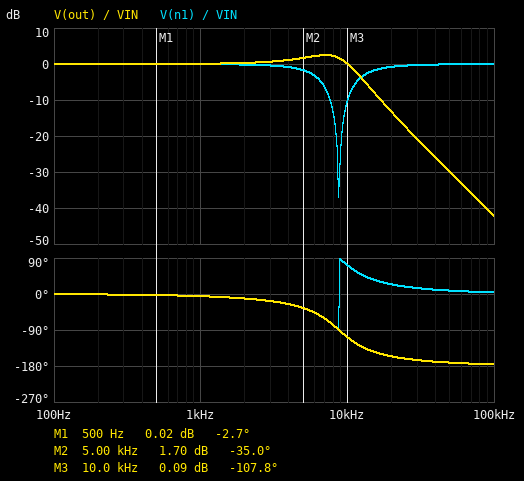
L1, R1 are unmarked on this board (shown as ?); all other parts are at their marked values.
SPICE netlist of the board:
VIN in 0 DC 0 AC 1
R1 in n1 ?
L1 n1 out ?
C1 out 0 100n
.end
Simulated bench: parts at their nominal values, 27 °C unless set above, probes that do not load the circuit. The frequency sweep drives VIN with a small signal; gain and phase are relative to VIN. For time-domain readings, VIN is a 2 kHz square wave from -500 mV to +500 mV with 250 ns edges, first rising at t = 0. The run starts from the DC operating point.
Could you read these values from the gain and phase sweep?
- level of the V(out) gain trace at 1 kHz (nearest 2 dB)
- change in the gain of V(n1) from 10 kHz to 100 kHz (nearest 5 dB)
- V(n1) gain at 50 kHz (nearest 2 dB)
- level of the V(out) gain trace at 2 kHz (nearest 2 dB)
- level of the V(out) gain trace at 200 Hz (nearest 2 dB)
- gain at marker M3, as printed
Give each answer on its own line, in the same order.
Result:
0 dB
10 dB
0 dB
0 dB
0 dB
0.09 dB
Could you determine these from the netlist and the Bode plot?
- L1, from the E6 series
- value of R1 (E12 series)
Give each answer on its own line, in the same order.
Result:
3.3 mH
150 Ω
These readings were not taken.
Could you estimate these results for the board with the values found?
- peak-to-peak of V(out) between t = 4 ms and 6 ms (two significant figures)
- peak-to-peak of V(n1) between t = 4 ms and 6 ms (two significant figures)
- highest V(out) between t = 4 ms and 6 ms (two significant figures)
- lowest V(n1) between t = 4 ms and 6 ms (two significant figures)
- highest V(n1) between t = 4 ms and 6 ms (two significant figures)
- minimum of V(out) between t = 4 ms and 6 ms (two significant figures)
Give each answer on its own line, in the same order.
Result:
1.5 V
1.2 V
740 mV
-620 mV
620 mV
-740 mV
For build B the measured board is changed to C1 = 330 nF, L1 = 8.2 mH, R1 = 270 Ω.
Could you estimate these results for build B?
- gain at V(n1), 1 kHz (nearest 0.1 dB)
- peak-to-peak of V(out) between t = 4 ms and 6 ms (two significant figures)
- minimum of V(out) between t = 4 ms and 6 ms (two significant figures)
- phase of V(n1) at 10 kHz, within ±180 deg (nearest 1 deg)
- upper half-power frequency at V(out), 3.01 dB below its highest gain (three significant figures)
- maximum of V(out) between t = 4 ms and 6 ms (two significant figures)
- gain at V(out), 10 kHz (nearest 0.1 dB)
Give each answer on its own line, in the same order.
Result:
-1.4 dB
990 mV
-500 mV
30 deg
2.44 kHz
500 mV
-21.0 dB
